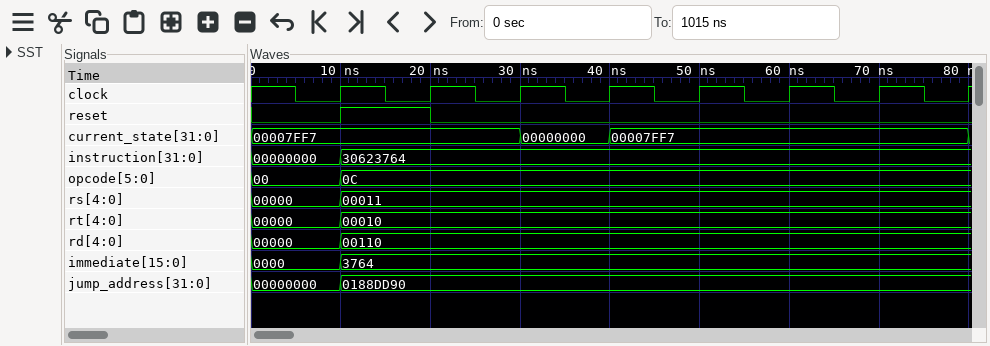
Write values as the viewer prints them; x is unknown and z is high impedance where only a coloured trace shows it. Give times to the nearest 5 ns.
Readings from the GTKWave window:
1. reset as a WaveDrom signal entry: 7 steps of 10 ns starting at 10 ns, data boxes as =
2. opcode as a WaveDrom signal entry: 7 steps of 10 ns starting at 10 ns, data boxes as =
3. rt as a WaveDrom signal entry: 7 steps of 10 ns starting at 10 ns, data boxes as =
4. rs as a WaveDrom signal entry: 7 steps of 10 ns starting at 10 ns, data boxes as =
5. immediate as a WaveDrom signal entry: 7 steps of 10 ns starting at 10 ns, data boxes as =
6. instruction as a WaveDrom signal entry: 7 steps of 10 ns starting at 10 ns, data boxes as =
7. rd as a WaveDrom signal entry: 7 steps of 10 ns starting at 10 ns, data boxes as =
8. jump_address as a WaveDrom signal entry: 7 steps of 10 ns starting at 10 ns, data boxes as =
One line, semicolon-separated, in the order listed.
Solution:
{name: 'reset', wave: '10.....'}; {name: 'opcode', wave: '=......', data: '0C'}; {name: 'rt', wave: '=......', data: '00010'}; {name: 'rs', wave: '=......', data: '00011'}; {name: 'immediate', wave: '=......', data: '3764'}; {name: 'instruction', wave: '=......', data: '30623764'}; {name: 'rd', wave: '=......', data: '00110'}; {name: 'jump_address', wave: '=......', data: '0188DD90'}
